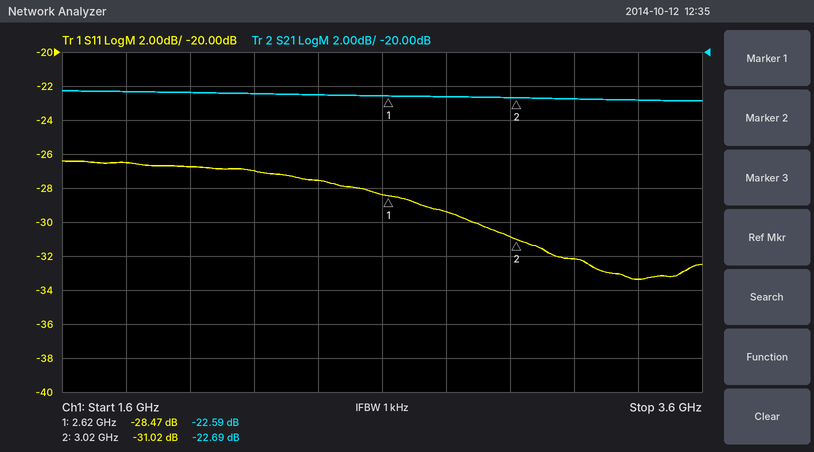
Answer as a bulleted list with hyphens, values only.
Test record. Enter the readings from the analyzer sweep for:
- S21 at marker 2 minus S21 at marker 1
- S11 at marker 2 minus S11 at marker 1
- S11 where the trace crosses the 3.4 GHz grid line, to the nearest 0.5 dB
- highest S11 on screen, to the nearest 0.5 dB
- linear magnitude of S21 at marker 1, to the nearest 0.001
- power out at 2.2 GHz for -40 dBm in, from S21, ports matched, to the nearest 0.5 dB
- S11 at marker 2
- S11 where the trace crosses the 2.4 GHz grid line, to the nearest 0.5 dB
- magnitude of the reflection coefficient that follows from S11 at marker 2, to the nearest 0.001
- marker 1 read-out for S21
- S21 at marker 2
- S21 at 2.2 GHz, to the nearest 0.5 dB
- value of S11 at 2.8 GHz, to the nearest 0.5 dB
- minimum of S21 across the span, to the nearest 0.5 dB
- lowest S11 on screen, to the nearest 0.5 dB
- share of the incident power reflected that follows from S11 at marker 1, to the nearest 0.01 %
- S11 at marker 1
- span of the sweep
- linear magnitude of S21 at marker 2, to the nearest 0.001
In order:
- -0.10 dB
- -2.55 dB
- -33.5 dB
- -26.5 dB
- 0.074
- -62.5 dBm
- -31.02 dB
- -27.5 dB
- 0.028
- -22.59 dB
- -22.69 dB
- -22.5 dB
- -29.5 dB
- -23.0 dB
- -33.5 dB
- 0.14 %
- -28.47 dB
- 2 GHz
- 0.073
